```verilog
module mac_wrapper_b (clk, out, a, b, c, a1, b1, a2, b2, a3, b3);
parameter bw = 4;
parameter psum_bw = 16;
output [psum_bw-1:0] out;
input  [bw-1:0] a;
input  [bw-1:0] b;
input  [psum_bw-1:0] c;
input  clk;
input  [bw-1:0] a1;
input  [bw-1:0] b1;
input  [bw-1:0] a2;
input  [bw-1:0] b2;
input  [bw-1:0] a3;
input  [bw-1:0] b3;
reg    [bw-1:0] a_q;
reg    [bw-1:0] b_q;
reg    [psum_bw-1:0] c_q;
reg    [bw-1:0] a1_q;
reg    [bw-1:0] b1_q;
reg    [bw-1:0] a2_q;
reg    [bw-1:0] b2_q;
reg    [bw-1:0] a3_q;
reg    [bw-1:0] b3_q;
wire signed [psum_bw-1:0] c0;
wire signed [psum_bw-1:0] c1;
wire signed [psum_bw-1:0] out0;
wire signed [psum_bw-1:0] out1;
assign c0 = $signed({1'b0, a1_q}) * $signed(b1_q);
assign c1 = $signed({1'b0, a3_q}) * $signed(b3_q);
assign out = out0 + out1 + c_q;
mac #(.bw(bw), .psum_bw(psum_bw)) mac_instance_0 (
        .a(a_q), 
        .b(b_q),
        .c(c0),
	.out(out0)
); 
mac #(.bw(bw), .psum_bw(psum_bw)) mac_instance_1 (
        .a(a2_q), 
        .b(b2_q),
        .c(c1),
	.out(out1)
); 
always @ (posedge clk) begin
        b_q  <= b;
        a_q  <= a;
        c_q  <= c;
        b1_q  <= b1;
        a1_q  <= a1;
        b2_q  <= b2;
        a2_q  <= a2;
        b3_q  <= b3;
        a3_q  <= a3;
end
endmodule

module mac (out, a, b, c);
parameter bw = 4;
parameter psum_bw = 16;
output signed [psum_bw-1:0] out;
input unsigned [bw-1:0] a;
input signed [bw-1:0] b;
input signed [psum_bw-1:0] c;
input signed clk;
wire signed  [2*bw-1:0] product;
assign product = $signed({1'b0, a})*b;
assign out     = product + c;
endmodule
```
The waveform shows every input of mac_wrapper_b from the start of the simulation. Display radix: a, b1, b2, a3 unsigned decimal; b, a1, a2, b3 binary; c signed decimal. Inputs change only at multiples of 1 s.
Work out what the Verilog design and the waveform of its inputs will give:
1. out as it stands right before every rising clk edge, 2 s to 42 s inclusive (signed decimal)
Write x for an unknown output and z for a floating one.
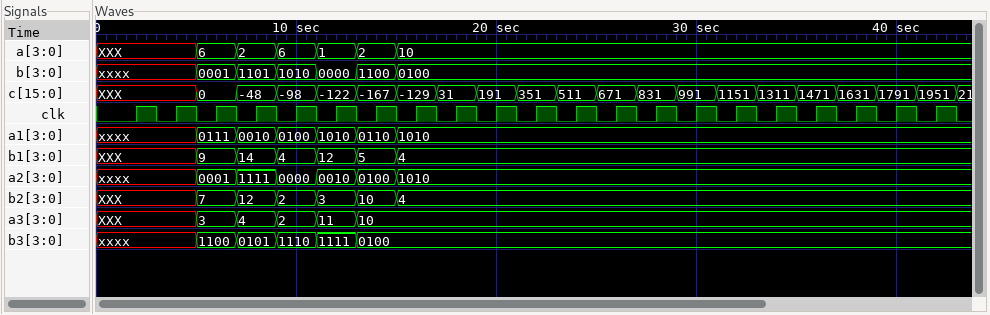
x, x, x, -48, -98, -122, -167, -129, 31, 191, 351, 511, 671, 831, 991, 1151, 1311, 1471, 1631, 1791, 1951
